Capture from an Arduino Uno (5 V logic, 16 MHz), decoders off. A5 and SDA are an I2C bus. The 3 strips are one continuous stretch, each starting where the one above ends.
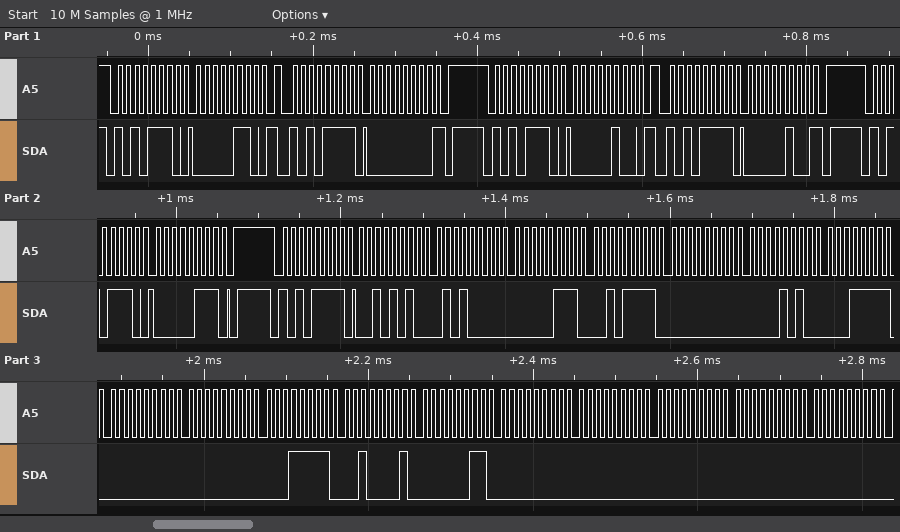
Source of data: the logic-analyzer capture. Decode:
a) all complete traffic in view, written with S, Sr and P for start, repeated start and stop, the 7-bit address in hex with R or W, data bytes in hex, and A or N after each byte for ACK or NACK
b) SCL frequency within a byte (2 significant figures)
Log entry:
S 57W A 06 A Sr 57R A 00 N P S 57W A 04 A Sr 57R A 04 N P S 57W A 07 A P S 57R A 2A A 50 A 07 A 2F A 00 A 0A A 1F A 00 A 00 A 1F A 21 A 03 A 00 A 00 A 00 A 00 A 00 A
100 kHz
